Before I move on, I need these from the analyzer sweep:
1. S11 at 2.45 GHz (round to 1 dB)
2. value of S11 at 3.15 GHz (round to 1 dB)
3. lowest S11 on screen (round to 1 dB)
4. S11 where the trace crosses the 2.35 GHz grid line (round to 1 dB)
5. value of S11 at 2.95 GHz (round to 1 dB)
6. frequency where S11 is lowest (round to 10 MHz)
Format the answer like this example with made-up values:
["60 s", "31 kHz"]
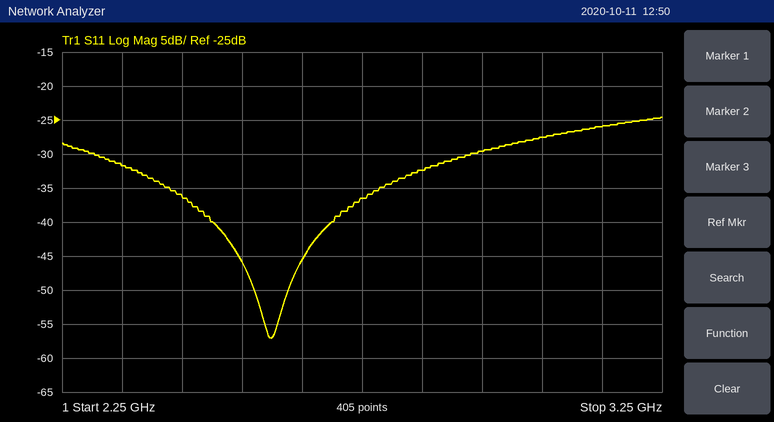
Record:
["-36 dB", "-26 dB", "-57 dB", "-32 dB", "-30 dB", "2.60 GHz"]
